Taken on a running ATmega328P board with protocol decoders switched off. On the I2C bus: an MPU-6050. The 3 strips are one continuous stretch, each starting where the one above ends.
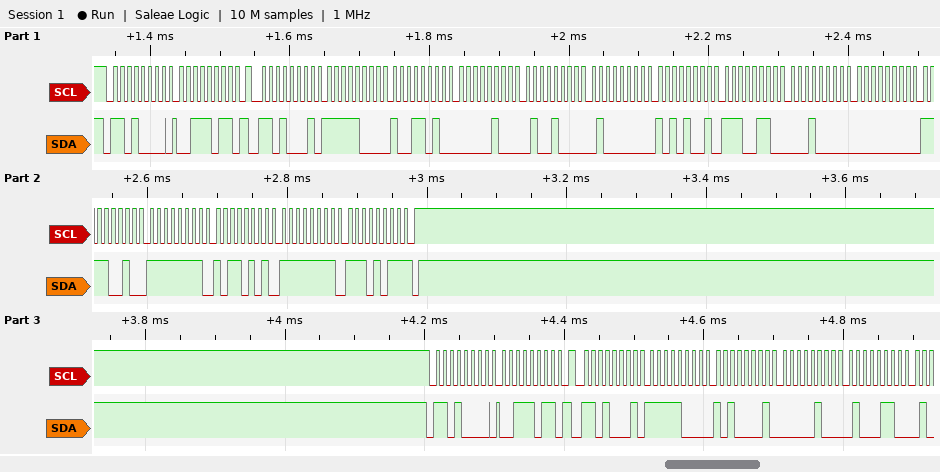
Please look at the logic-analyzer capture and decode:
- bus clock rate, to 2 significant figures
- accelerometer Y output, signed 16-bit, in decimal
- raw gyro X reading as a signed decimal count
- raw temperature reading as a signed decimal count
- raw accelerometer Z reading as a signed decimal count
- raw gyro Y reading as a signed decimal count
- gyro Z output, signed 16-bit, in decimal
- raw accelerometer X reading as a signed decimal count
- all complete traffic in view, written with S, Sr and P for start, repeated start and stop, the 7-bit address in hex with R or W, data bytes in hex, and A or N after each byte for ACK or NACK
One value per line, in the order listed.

100 kHz
1096
242
-6640
16553
-75
-21
-1894
S 68W A 3B A Sr 68R A F8 A 9A A 04 A 48 A 40 A A9 A E6 A 10 A 00 A F2 A FF A B5 A FF A EB N P S 68W A 3B A Sr 68R A F8 A A1 A 04 A 46 A
